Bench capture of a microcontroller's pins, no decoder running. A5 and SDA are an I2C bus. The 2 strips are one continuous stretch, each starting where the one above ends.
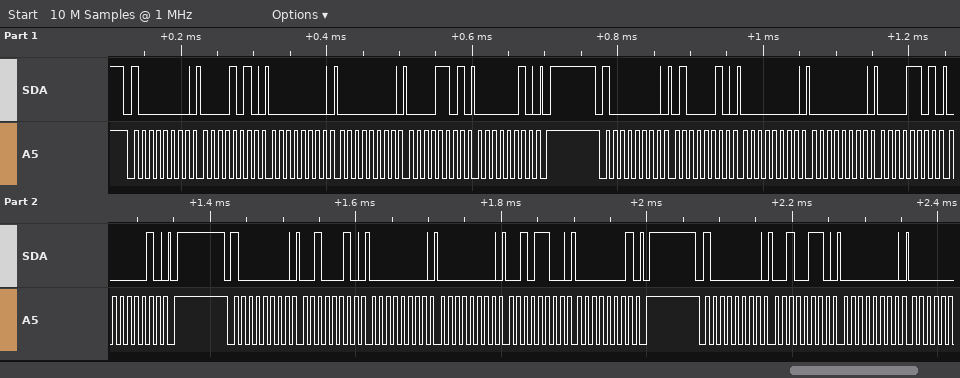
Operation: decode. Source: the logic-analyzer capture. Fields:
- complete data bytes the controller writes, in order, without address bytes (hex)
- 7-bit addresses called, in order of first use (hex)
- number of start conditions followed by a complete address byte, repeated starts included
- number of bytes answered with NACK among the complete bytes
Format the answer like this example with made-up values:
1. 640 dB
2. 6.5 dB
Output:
1. 0A 00 00 0D 02 42 00 00 0D 02 22 00 00 2C 01 26 00
2. 0x40
3. 4
4. 0
